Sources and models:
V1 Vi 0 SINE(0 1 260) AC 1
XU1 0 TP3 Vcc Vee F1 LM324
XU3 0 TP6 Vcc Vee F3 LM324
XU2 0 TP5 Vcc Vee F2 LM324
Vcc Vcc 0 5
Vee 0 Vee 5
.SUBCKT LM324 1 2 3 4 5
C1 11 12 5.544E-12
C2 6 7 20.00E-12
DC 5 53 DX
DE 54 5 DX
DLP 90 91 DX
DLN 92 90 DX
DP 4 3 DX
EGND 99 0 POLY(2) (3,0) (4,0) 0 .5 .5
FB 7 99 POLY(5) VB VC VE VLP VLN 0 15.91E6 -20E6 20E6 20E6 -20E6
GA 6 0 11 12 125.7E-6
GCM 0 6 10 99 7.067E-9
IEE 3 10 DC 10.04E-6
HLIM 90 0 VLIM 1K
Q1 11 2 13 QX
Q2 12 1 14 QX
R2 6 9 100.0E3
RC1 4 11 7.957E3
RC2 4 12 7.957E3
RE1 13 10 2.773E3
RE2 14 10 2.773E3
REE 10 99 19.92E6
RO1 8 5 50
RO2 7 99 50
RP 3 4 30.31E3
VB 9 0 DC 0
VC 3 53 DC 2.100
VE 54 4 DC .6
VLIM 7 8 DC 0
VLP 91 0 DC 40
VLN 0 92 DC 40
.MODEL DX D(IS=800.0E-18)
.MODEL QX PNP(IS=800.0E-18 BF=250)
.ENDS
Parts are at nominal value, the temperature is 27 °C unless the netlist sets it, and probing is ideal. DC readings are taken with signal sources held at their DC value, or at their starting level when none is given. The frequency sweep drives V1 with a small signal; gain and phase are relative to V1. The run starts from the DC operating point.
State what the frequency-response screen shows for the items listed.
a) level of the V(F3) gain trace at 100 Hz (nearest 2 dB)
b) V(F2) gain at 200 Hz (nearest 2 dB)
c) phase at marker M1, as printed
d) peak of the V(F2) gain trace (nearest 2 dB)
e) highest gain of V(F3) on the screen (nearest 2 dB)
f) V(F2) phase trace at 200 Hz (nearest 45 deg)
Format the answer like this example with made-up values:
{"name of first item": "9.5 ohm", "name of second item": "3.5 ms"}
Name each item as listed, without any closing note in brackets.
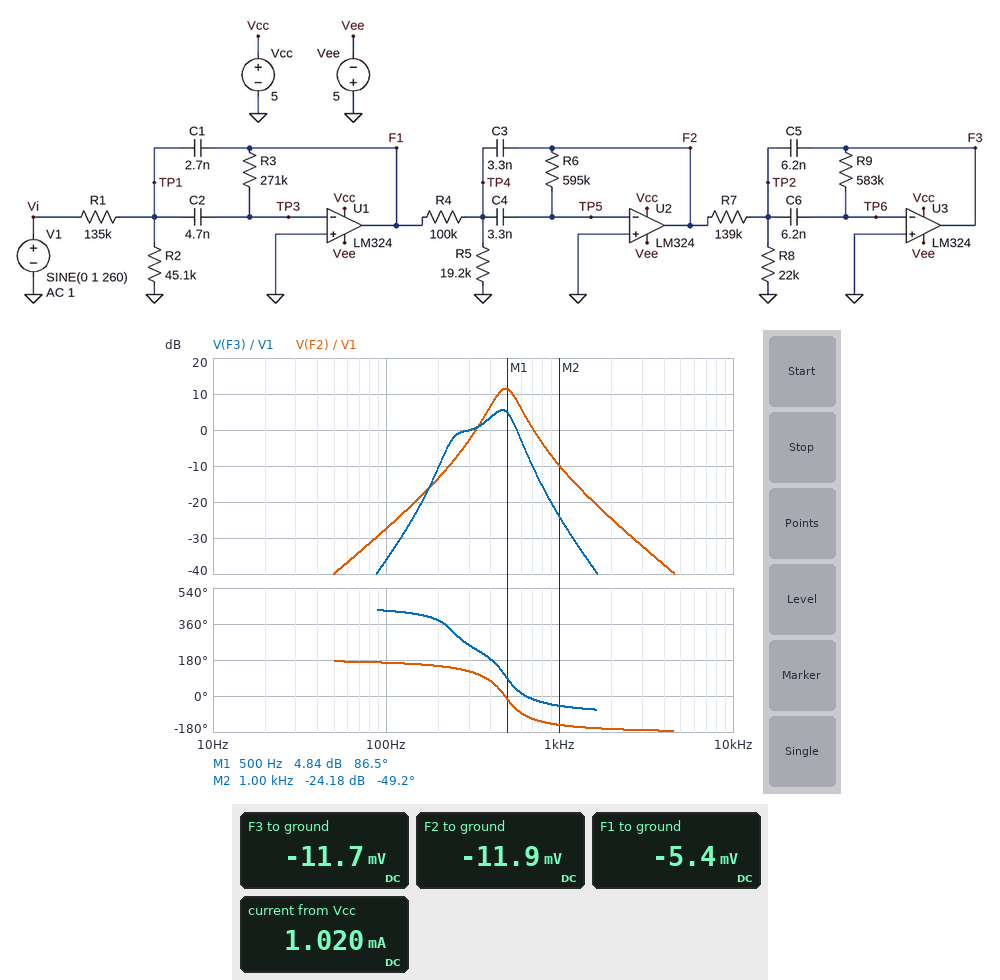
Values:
{"level of the V(F3) gain trace at 100 Hz": "-36 dB", "V(F2) gain at 200 Hz": "-14 dB", "phase at marker M1, as printed": "86.5 deg", "peak of the V(F2) gain trace": "12 dB", "highest gain of V(F3) on the screen": "6 dB", "V(F2) phase trace at 200 Hz": "135 deg"}
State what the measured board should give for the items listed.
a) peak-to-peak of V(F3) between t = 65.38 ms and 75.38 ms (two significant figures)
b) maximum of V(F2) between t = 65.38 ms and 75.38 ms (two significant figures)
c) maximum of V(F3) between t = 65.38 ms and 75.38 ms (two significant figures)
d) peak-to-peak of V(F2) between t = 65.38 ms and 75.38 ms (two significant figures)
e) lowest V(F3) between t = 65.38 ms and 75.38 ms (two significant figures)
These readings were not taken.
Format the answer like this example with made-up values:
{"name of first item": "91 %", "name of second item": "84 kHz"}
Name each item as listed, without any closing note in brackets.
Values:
{"peak-to-peak of V(F3) between t = 65.38 ms and 75.38 ms": "1.8 V", "maximum of V(F2) between t = 65.38 ms and 75.38 ms": "440 mV", "maximum of V(F3) between t = 65.38 ms and 75.38 ms": "880 mV", "peak-to-peak of V(F2) between t = 65.38 ms and 75.38 ms": "910 mV", "lowest V(F3) between t = 65.38 ms and 75.38 ms": "-910 mV"}
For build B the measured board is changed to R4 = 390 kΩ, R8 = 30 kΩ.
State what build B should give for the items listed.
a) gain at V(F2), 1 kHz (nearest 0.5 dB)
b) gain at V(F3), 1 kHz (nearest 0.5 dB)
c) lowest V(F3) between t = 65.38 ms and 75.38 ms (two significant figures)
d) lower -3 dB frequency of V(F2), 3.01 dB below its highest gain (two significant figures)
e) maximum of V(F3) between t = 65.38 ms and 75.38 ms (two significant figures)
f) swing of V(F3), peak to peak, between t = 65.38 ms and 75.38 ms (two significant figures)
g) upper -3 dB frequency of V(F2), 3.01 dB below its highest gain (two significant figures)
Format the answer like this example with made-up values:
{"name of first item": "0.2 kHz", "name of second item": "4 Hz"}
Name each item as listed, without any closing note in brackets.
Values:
{"gain at V(F2), 1 kHz": "-22.0 dB", "gain at V(F3), 1 kHz": "-36.5 dB", "lowest V(F3) between t = 65.38 ms and 75.38 ms": "-220 mV", "lower -3 dB frequency of V(F2), 3.01 dB below its highest gain": "400 Hz", "maximum of V(F3) between t = 65.38 ms and 75.38 ms": "200 mV", "swing of V(F3), peak to peak, between t = 65.38 ms and 75.38 ms": "420 mV", "upper -3 dB frequency of V(F2), 3.01 dB below its highest gain": "540 Hz"}
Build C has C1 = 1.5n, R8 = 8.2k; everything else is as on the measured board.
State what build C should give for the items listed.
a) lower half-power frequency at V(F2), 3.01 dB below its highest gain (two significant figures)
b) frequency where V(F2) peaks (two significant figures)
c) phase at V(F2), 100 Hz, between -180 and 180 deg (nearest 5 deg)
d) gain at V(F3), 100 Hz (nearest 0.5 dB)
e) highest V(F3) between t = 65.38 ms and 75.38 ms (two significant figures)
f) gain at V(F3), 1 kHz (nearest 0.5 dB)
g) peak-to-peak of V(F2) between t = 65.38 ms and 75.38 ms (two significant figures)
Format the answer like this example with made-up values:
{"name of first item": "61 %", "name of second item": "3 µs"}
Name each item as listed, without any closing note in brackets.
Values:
{"lower half-power frequency at V(F2), 3.01 dB below its highest gain": "440 Hz", "frequency where V(F2) peaks": "510 Hz", "phase at V(F2), 100 Hz, between -180 and 180 deg": "170 deg", "gain at V(F3), 100 Hz": "-45.0 dB", "highest V(F3) between t = 65.38 ms and 75.38 ms": "230 mV", "gain at V(F3), 1 kHz": "-17.5 dB", "peak-to-peak of V(F2) between t = 65.38 ms and 75.38 ms": "810 mV"}
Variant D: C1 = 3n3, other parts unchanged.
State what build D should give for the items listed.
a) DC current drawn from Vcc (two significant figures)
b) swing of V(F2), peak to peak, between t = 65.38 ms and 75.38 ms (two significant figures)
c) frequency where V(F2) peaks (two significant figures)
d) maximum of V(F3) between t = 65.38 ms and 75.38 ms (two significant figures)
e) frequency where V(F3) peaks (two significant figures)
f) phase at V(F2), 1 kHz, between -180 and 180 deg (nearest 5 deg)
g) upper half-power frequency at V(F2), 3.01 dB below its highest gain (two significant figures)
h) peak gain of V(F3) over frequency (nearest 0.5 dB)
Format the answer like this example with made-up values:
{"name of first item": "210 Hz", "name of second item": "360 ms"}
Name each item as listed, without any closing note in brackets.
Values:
{"DC current drawn from Vcc": "1.0 mA", "swing of V(F2), peak to peak, between t = 65.38 ms and 75.38 ms": "950 mV", "frequency where V(F2) peaks": "480 Hz", "maximum of V(F3) between t = 65.38 ms and 75.38 ms": "930 mV", "frequency where V(F3) peaks": "460 Hz", "phase at V(F2), 1 kHz, between -180 and 180 deg": "-150 deg", "upper half-power frequency at V(F2), 3.01 dB below its highest gain": "550 Hz", "peak gain of V(F3) over frequency": "4.5 dB"}
